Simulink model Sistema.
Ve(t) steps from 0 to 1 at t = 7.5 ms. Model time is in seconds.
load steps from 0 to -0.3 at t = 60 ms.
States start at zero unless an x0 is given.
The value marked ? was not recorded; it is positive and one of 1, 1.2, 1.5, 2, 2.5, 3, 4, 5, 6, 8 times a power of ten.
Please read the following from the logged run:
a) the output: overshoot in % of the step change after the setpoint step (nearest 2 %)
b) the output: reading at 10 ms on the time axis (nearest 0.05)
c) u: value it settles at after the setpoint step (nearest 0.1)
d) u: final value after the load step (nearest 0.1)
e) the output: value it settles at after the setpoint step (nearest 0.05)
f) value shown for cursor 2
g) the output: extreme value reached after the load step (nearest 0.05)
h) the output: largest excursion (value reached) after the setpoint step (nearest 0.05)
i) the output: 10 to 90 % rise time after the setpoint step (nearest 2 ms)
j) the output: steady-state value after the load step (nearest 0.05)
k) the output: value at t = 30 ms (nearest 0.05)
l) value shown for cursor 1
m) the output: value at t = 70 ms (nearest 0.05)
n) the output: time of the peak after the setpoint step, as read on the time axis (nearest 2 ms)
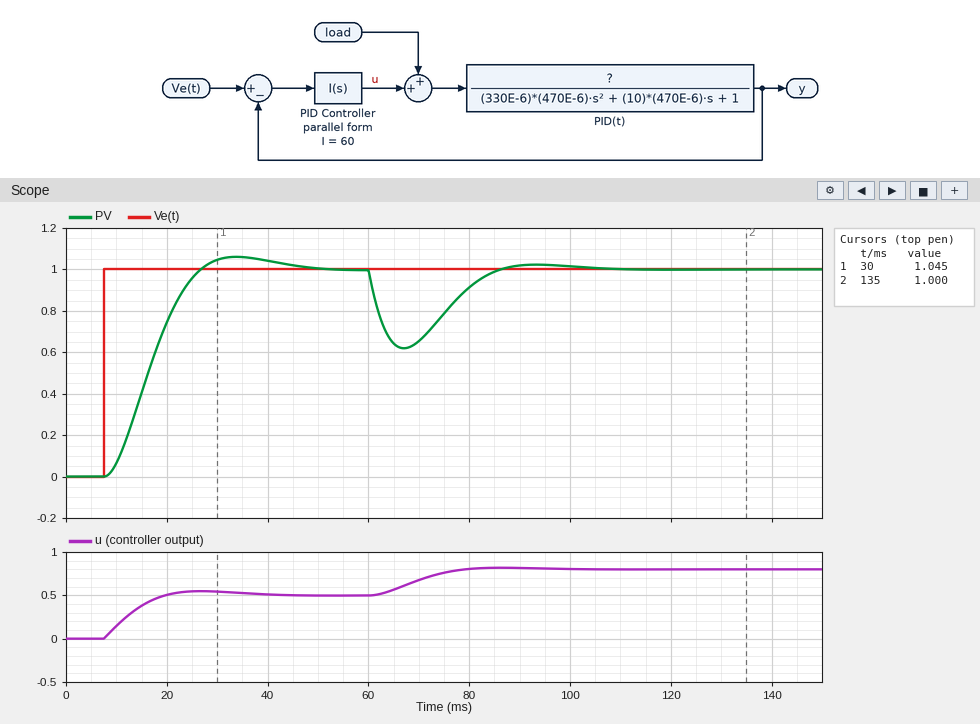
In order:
6 %
0.05
0.5
0.8
1.00
1.000
0.60
1.05
12 ms
1.00
1.05
1.045
0.65
34 ms
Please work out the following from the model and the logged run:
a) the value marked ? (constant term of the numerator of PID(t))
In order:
2
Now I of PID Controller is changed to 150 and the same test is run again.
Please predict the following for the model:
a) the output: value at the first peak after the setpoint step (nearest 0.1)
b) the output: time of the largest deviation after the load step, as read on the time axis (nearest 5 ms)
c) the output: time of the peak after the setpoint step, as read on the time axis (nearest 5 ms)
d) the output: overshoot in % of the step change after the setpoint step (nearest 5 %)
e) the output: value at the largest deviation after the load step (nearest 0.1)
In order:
1.2
65 ms
20 ms
25 %
0.7
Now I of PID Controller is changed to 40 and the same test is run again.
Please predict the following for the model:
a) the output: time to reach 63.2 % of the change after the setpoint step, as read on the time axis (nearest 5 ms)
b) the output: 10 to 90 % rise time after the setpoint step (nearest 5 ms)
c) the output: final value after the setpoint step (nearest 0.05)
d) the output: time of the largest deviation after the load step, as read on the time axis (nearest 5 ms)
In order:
20 ms
20 ms
1.00
70 ms
